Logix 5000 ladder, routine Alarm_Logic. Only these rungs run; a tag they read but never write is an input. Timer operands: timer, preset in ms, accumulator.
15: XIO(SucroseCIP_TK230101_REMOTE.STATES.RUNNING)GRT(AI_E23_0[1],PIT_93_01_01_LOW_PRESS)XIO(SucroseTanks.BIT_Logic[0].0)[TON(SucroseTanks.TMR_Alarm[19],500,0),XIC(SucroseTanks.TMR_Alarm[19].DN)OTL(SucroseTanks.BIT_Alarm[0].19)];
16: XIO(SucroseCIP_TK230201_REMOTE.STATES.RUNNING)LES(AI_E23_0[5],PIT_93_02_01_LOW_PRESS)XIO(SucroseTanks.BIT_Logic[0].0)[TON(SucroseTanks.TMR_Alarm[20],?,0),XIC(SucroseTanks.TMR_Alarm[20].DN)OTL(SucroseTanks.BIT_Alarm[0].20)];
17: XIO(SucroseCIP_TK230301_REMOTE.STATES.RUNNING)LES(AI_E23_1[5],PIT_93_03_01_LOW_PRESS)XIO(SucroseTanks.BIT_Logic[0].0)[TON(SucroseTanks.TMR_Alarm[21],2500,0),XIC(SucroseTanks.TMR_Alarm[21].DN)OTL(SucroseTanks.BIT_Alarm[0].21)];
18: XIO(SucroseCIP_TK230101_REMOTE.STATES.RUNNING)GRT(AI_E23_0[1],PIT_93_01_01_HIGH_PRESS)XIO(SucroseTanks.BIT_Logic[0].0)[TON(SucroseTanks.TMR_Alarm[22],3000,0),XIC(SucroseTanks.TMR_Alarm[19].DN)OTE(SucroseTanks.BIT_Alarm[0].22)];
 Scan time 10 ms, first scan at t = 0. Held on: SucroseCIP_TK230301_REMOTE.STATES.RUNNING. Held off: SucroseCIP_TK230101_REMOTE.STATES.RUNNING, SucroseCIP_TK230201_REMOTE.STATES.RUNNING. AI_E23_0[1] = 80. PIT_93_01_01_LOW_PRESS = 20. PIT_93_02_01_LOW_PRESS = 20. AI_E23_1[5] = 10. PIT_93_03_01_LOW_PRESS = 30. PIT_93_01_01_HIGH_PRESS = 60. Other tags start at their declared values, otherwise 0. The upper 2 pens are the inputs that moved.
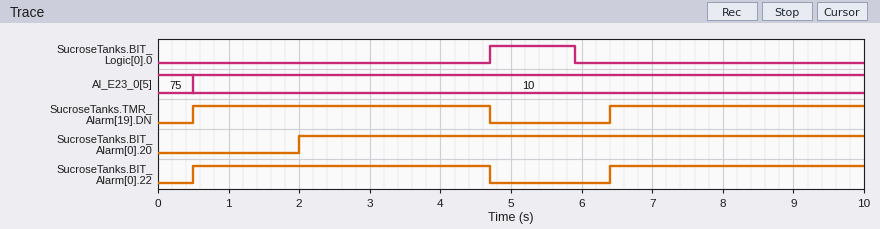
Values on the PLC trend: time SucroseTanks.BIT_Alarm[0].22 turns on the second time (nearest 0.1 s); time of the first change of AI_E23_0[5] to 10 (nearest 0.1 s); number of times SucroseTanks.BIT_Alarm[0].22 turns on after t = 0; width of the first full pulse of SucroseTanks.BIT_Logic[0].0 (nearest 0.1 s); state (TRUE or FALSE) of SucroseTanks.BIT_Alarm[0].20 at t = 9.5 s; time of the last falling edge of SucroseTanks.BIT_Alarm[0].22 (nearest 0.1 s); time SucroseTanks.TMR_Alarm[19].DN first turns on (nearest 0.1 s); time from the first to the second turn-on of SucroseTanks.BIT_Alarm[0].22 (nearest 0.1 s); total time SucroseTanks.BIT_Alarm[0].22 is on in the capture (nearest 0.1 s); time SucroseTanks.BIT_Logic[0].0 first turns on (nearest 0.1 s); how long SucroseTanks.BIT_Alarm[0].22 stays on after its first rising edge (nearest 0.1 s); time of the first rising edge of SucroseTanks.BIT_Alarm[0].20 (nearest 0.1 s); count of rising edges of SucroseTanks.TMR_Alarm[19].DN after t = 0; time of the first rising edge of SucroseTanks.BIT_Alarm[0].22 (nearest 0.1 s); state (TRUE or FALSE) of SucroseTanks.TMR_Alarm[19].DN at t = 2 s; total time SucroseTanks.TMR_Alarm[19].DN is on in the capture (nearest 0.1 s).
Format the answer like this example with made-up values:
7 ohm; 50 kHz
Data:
6.4 s; 0.5 s; 2; 1.2 s; TRUE; 4.7 s; 0.5 s; 5.9 s; 7.8 s; 4.7 s; 4.2 s; 2.0 s; 2; 0.5 s; TRUE; 7.8 s
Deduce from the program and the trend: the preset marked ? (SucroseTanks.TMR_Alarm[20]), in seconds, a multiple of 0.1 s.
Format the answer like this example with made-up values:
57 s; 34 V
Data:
1.5 s
